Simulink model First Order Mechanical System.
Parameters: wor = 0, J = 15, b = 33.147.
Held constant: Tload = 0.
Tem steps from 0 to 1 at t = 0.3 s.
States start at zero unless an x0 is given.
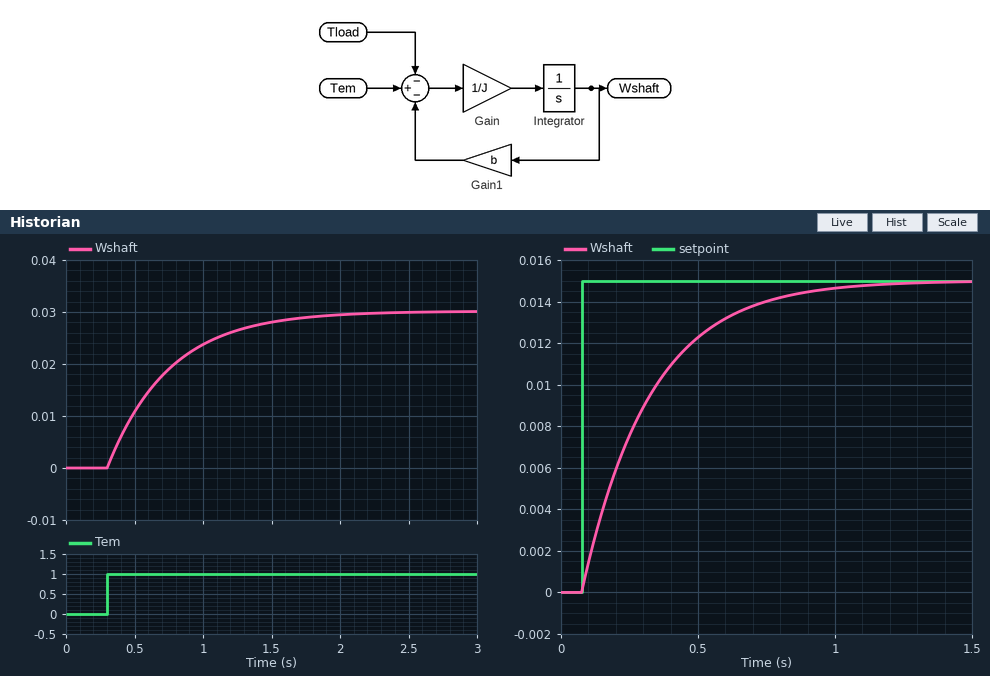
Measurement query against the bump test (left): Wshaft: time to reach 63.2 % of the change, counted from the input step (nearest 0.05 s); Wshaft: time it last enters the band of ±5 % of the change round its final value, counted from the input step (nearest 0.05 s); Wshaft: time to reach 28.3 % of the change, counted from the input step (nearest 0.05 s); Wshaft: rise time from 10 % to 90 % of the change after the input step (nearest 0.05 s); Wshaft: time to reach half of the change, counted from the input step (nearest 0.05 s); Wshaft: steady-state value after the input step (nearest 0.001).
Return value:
0.45 s
1.35 s
0.15 s
1.00 s
0.30 s
0.030
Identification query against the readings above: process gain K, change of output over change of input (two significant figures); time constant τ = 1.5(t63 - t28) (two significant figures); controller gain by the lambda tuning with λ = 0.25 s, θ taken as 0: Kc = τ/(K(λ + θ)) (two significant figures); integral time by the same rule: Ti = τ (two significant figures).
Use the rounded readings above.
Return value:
0.030
0.45 s
60
0.45 s
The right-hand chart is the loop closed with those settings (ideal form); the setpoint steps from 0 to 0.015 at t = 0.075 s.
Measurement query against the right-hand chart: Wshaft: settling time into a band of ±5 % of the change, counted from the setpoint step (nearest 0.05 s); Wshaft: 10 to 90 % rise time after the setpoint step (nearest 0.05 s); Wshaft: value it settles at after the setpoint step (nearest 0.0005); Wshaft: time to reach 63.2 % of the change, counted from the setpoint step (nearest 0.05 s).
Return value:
0.75 s
0.55 s
0.0150
0.25 s
